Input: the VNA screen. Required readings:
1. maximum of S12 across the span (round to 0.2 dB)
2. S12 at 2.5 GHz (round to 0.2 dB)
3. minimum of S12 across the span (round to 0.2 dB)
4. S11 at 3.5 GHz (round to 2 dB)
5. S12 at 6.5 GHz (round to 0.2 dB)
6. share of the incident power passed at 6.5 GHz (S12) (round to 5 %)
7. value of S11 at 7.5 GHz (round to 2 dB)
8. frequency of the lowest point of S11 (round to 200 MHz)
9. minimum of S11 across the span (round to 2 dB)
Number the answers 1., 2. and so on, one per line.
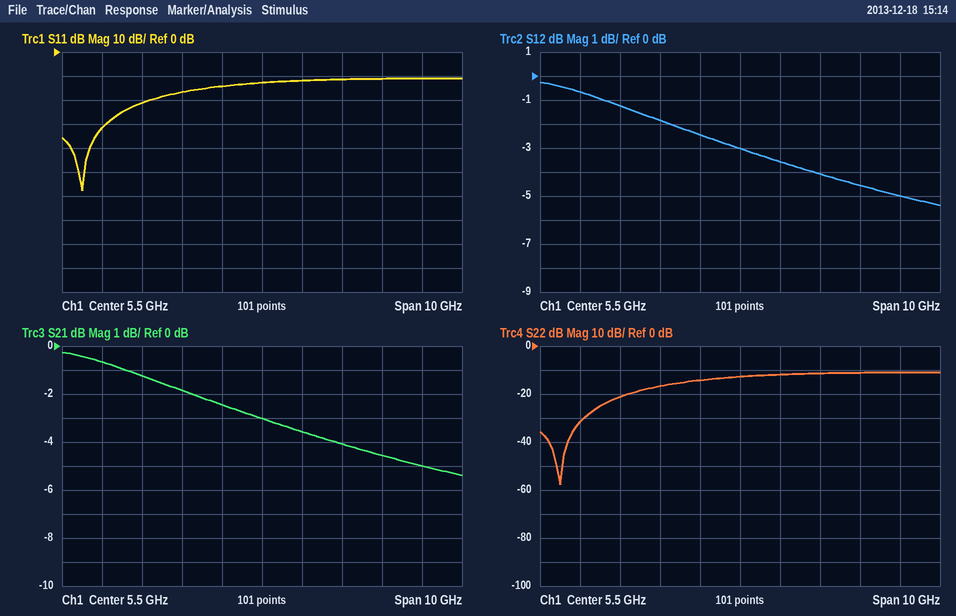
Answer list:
1. -0.2 dB
2. -1.2 dB
3. -5.4 dB
4. -16 dB
5. -3.6 dB
6. 45 %
7. -12 dB
8. 1.0 GHz
9. -58 dB
